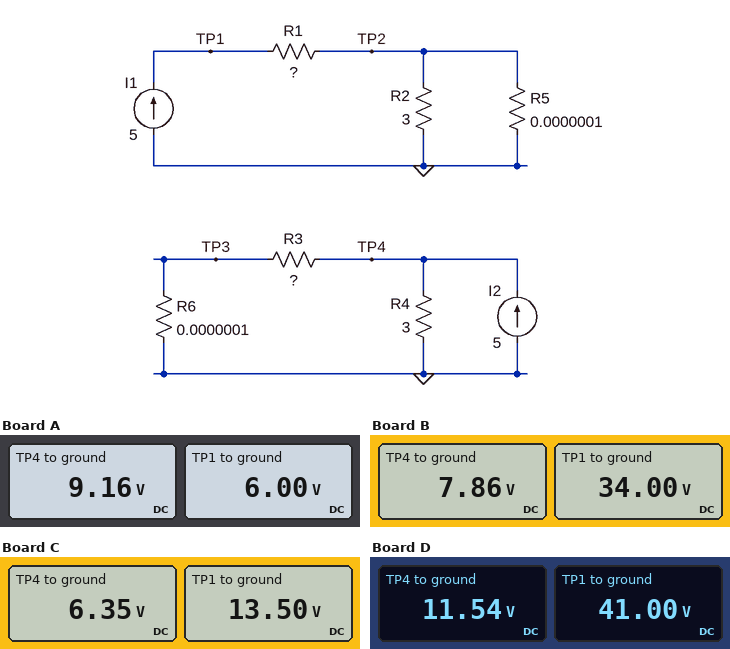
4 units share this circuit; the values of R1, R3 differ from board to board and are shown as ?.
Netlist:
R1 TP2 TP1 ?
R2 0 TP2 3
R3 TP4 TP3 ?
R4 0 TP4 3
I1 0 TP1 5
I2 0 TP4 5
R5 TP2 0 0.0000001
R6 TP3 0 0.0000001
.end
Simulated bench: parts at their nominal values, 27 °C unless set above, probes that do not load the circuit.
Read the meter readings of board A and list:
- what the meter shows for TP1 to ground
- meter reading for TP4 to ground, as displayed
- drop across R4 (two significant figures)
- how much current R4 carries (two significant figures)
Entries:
6.00 V
9.16 V
9.2 V
3.1 A
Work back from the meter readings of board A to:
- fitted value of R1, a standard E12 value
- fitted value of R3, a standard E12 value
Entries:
1.2 Ω
4.7 Ω
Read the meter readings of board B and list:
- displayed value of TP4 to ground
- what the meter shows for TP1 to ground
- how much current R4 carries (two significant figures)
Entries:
7.86 V
34.00 V
2.6 A
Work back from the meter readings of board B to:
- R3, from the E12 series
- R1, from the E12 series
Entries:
3.3 Ω
6.8 Ω
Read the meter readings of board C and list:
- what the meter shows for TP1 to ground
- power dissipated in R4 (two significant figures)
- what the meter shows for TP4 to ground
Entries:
13.50 V
13 W
6.35 V
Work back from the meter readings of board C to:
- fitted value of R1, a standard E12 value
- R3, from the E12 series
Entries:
2.7 Ω
2.2 Ω
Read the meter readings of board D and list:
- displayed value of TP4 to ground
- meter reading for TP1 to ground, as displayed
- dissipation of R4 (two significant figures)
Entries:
11.54 V
41.00 V
44 W
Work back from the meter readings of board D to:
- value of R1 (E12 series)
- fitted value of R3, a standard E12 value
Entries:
8.2 Ω
10 Ω
